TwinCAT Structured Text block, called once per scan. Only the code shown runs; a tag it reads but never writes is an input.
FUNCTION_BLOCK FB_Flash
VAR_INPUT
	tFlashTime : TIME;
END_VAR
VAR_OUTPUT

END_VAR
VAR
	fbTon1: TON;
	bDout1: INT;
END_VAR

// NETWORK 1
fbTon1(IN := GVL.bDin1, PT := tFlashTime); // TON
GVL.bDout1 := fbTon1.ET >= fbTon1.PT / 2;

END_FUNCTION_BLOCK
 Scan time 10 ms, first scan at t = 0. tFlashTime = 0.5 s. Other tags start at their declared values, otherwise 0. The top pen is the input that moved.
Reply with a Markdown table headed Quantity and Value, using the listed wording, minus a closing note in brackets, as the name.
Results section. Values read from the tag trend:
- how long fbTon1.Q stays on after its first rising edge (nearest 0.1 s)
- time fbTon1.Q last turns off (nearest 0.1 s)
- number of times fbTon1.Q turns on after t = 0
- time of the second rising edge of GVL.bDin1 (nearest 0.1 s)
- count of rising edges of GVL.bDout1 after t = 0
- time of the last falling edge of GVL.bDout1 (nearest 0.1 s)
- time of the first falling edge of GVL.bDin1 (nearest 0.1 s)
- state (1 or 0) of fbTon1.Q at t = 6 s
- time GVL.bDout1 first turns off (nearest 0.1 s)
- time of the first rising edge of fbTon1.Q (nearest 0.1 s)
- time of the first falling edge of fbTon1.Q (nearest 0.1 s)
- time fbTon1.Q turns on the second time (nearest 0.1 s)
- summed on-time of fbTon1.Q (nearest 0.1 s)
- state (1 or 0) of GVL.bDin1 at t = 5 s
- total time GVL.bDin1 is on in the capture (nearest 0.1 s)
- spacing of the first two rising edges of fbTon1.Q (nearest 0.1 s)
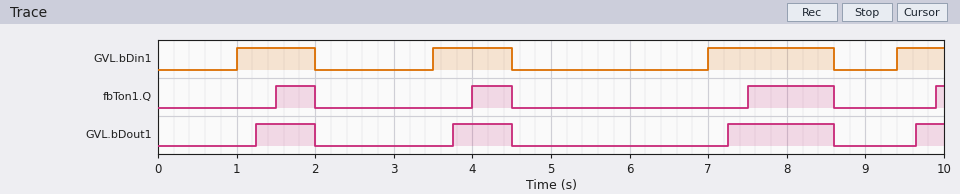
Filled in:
| Quantity | Value |
|---|---|
| how long fbTon1.Q stays on after its first rising edge | 0.5 s |
| time fbTon1.Q last turns off | 8.6 s |
| number of times fbTon1.Q turns on after t = 0 | 4 |
| time of the second rising edge of GVL.bDin1 | 3.5 s |
| count of rising edges of GVL.bDout1 after t = 0 | 4 |
| time of the last falling edge of GVL.bDout1 | 8.6 s |
| time of the first falling edge of GVL.bDin1 | 2.0 s |
| state (1 or 0) of fbTon1.Q at t = 6 s | 0 |
| time GVL.bDout1 first turns off | 2.0 s |
| time of the first rising edge of fbTon1.Q | 1.5 s |
| time of the first falling edge of fbTon1.Q | 2.0 s |
| time fbTon1.Q turns on the second time | 4.0 s |
| summed on-time of fbTon1.Q | 2.2 s |
| state (1 or 0) of GVL.bDin1 at t = 5 s | 0 |
| total time GVL.bDin1 is on in the capture | 4.2 s |
| spacing of the first two rising edges of fbTon1.Q | 2.5 s |
